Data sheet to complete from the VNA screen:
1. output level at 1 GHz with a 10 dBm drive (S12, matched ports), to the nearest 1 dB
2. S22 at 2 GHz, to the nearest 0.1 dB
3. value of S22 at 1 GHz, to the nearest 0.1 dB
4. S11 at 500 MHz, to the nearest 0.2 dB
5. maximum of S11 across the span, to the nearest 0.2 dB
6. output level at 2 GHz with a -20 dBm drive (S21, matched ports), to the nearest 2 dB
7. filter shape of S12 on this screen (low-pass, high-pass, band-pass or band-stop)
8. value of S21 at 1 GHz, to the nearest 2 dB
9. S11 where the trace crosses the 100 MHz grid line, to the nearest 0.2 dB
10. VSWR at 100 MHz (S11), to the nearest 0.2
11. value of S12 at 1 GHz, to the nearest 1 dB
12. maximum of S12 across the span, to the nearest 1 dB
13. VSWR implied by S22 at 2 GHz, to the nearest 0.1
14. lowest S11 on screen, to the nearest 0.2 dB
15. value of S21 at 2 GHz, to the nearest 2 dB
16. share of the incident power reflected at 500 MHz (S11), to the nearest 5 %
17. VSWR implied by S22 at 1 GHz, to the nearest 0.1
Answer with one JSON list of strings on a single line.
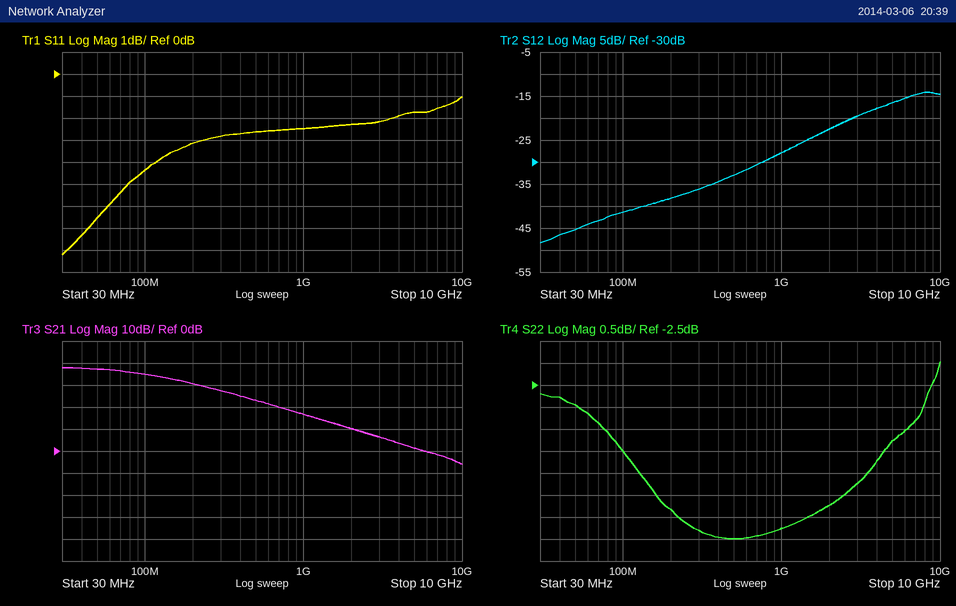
["-18 dBm", "-5.2 dB", "-5.8 dB", "-2.6 dB", "-1.0 dB", "-10 dBm", "high-pass", "16 dB", "-4.4 dB", "4.0", "-28 dB", "-14 dB", "3.4", "-8.2 dB", "10 dB", "55 %", "3.1"]
